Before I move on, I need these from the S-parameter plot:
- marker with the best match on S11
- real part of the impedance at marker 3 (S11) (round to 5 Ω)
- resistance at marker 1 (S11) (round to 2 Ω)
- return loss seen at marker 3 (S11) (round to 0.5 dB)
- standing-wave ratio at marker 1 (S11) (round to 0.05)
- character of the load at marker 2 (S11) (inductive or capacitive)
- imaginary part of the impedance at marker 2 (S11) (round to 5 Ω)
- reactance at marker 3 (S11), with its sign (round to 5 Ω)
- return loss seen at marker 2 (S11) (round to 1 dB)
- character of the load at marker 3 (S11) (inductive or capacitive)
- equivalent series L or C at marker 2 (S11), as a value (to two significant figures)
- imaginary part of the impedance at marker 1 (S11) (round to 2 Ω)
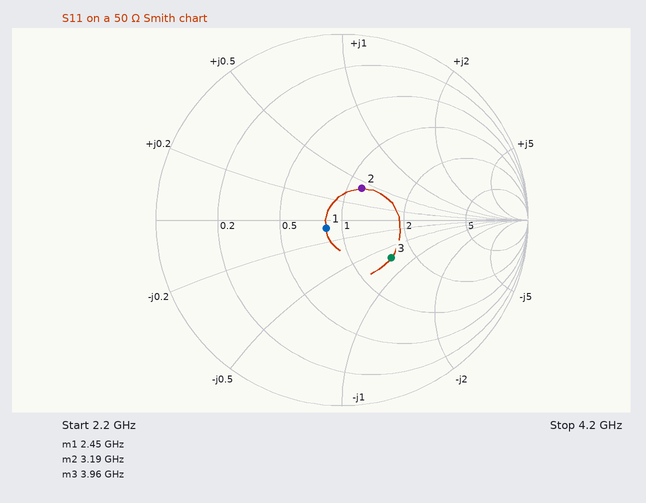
marker 1
75 Ω
42 Ω
9.5 dB
1.20
inductive
+20 Ω
-35 Ω
14 dB
capacitive
1.0 nH
-4 Ω
